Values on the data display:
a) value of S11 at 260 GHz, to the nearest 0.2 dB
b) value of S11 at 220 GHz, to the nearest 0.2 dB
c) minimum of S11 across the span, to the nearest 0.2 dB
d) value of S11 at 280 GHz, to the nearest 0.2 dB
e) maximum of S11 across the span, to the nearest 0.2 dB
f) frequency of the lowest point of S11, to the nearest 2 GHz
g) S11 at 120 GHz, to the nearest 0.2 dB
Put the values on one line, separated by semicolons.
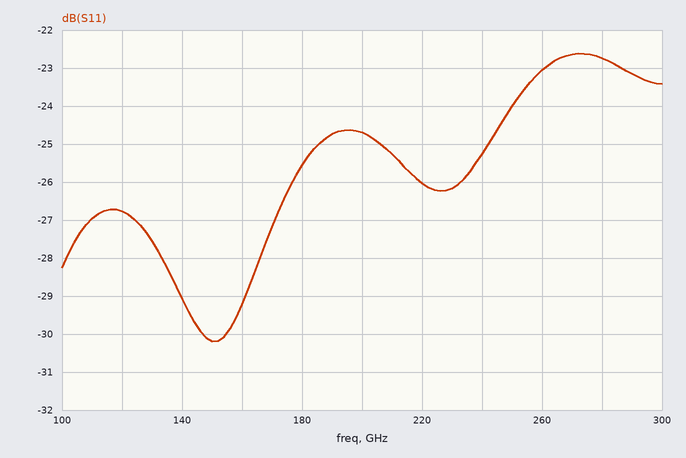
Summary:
-23.0 dB; -26.0 dB; -30.2 dB; -22.8 dB; -22.6 dB; 150 GHz; -26.8 dB
